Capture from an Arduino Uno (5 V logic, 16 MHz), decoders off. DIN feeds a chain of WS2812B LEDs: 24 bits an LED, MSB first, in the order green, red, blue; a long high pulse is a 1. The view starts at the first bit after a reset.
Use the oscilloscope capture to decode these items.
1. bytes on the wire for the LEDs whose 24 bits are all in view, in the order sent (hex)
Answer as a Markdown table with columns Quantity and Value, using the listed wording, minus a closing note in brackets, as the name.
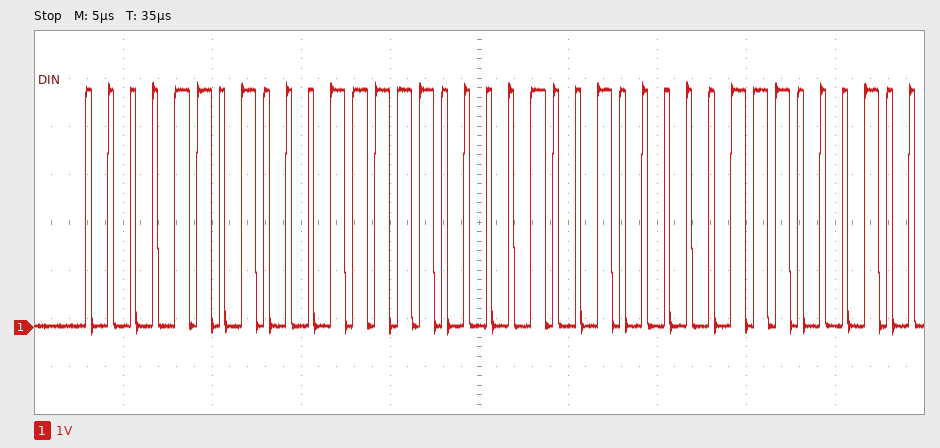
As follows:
| Quantity | Value |
|---|---|
| bytes on the wire for the LEDs whose 24 bits are all in view, in the order sent | 0D 1F 09 |
